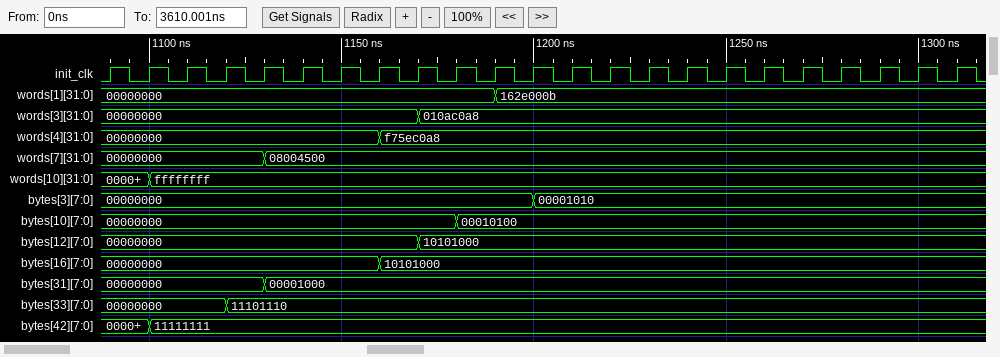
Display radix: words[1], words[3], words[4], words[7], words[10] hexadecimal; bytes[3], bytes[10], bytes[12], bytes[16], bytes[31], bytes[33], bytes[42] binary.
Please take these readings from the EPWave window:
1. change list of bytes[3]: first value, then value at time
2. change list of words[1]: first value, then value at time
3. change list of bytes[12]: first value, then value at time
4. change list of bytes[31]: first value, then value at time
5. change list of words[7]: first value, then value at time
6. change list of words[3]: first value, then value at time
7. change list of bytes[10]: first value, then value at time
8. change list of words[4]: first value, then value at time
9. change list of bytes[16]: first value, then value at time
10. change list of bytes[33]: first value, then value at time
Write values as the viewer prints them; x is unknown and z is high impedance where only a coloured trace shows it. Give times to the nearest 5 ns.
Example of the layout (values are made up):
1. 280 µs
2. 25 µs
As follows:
1. 00000000, 00001010 at 1200 ns
2. 00000000, 162e000b at 1190 ns
3. 00000000, 10101000 at 1170 ns
4. 00000000, 00001000 at 1130 ns
5. 00000000, 08004500 at 1130 ns
6. 00000000, 010ac0a8 at 1170 ns
7. 00000000, 00010100 at 1180 ns
8. 00000000, f75ec0a8 at 1160 ns
9. 00000000, 10101000 at 1160 ns
10. 00000000, 11101110 at 1120 ns
